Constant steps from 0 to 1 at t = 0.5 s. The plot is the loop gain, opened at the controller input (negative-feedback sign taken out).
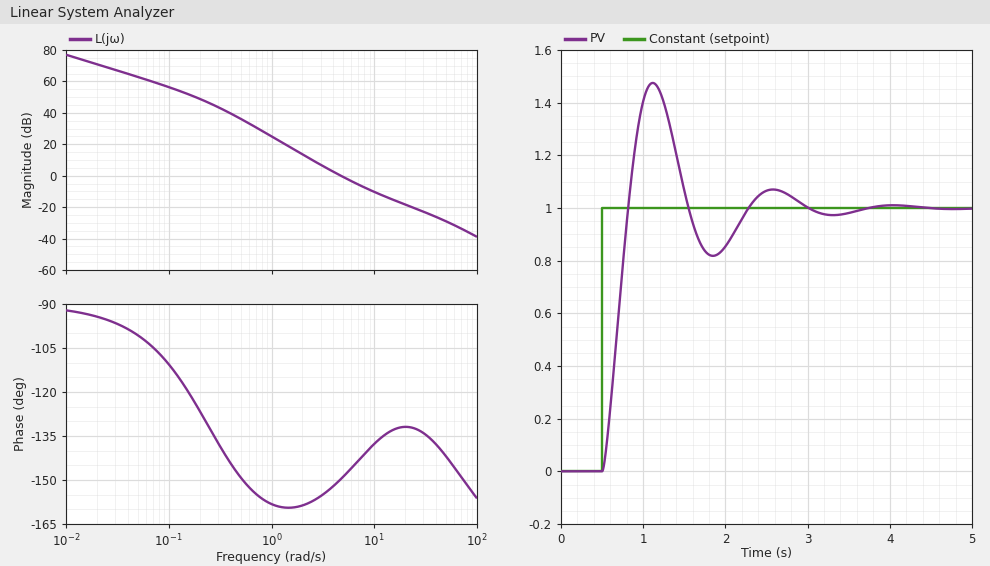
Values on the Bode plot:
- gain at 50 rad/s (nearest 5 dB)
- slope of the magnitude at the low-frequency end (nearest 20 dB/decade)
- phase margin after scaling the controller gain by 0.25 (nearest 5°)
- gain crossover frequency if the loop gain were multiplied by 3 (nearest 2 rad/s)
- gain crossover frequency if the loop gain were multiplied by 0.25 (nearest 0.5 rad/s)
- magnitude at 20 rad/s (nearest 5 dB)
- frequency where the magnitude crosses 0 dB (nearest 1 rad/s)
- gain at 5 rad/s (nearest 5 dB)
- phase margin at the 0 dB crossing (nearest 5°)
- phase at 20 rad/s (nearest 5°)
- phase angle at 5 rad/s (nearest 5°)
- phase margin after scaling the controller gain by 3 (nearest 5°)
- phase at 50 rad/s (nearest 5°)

-30 dB
-20 dB/decade
20°
10 rad/s
2.0 rad/s
-20 dB
5 rad/s
0 dB
30°
-130°
-150°
40°
-140°
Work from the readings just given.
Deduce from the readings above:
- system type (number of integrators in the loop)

1
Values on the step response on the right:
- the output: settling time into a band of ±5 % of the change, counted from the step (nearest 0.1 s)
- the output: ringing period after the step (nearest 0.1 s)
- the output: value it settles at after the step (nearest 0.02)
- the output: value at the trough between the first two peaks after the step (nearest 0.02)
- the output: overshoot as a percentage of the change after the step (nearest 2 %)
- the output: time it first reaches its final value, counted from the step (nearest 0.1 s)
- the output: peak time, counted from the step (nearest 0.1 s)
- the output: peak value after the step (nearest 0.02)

2.3 s
1.5 s
1.00
0.82
48 %
0.3 s
0.6 s
1.48
